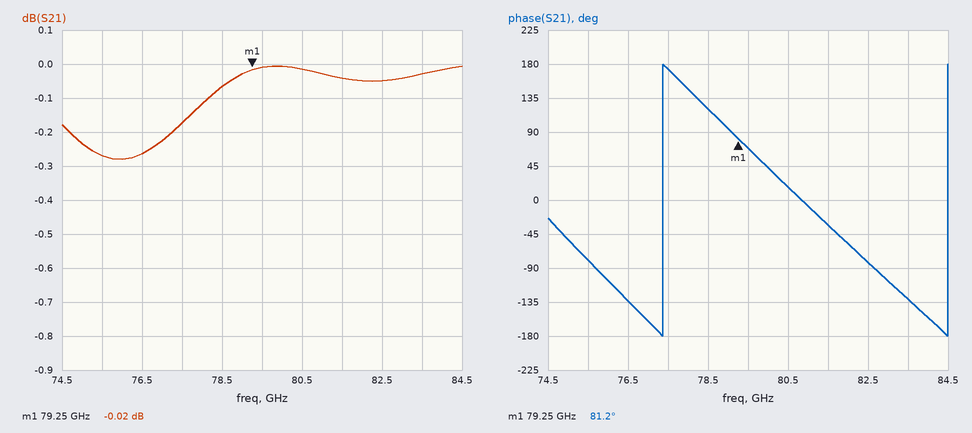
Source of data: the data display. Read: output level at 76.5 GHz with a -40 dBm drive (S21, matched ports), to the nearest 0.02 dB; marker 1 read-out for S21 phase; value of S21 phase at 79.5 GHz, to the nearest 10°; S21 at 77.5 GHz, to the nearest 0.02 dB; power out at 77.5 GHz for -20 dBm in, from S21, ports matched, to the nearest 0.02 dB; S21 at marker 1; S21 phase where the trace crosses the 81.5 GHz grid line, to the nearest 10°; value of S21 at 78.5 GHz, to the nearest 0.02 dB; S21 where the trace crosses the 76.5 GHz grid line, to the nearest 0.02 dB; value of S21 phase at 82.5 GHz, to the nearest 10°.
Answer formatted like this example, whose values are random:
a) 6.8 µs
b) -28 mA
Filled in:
a) -40.26 dBm
b) 81.2°
c) 70°
d) -0.18 dB
e) -20.18 dBm
f) -0.02 dB
g) -30°
h) -0.06 dB
i) -0.26 dB
j) -80°
